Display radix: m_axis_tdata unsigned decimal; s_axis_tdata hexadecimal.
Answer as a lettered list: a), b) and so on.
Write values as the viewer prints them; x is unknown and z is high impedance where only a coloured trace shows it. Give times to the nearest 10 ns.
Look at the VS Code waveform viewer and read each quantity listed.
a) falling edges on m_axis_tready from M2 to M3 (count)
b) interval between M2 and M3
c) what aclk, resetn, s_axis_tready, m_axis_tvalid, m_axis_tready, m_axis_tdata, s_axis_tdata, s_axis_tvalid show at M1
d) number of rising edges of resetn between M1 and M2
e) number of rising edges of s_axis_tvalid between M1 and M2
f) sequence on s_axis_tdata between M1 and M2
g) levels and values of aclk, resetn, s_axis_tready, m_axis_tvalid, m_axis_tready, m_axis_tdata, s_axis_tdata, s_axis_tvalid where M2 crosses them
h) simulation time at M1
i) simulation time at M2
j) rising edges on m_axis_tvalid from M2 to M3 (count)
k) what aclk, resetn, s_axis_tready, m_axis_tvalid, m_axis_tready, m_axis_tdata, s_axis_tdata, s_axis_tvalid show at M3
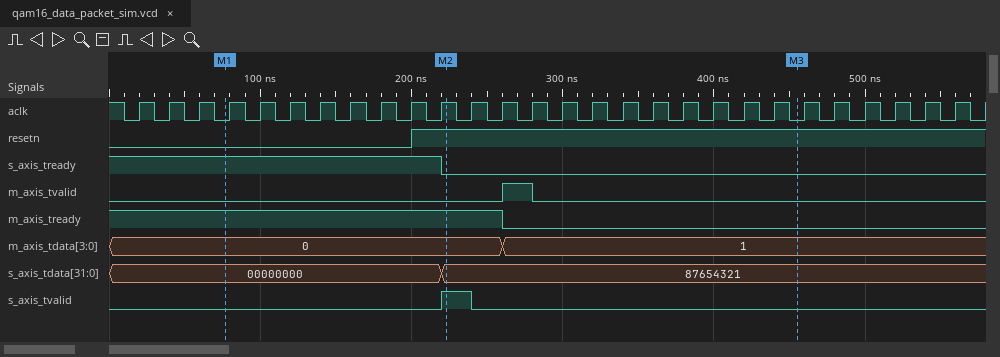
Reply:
a) 1
b) 230 ns
c) aclk=0, resetn=0, s_axis_tready=1, m_axis_tvalid=0, m_axis_tready=1, m_axis_tdata=0, s_axis_tdata=00000000, s_axis_tvalid=0
d) 1
e) 1
f) 00000000, 87654321
g) aclk=1, resetn=1, s_axis_tready=0, m_axis_tvalid=0, m_axis_tready=1, m_axis_tdata=0, s_axis_tdata=87654321, s_axis_tvalid=1
h) 80 ns
i) 220 ns
j) 1
k) aclk=0, resetn=1, s_axis_tready=0, m_axis_tvalid=0, m_axis_tready=0, m_axis_tdata=1, s_axis_tdata=87654321, s_axis_tvalid=0
